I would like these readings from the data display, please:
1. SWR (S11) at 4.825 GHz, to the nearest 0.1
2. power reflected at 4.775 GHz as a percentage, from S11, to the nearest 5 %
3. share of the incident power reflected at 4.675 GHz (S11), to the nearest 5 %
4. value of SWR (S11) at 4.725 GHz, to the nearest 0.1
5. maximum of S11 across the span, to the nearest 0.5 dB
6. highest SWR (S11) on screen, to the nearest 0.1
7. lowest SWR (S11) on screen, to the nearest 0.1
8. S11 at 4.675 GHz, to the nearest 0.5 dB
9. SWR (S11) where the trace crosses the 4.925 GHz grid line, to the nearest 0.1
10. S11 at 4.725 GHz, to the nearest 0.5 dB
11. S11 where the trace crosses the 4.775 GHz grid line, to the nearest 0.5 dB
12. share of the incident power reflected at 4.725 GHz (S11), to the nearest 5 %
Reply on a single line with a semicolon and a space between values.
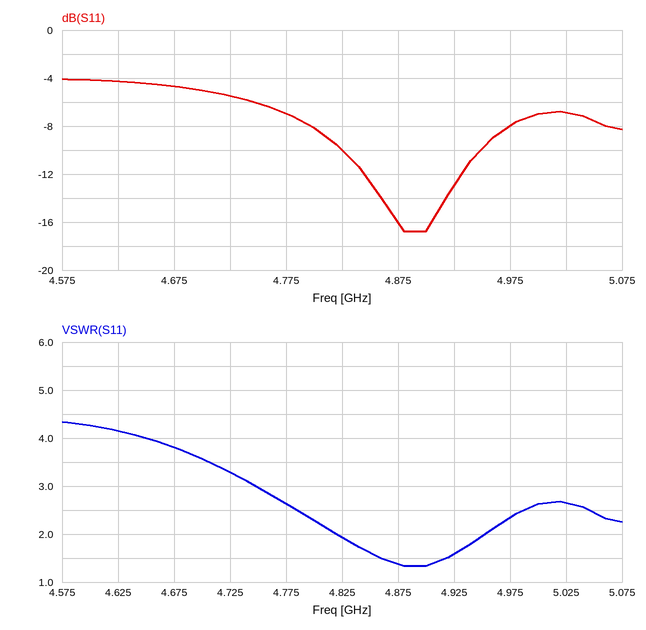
1.9; 20 %; 35 %; 3.3; -4.0 dB; 4.3; 1.3; -4.5 dB; 1.6; -5.5 dB; -7.0 dB; 30 %
